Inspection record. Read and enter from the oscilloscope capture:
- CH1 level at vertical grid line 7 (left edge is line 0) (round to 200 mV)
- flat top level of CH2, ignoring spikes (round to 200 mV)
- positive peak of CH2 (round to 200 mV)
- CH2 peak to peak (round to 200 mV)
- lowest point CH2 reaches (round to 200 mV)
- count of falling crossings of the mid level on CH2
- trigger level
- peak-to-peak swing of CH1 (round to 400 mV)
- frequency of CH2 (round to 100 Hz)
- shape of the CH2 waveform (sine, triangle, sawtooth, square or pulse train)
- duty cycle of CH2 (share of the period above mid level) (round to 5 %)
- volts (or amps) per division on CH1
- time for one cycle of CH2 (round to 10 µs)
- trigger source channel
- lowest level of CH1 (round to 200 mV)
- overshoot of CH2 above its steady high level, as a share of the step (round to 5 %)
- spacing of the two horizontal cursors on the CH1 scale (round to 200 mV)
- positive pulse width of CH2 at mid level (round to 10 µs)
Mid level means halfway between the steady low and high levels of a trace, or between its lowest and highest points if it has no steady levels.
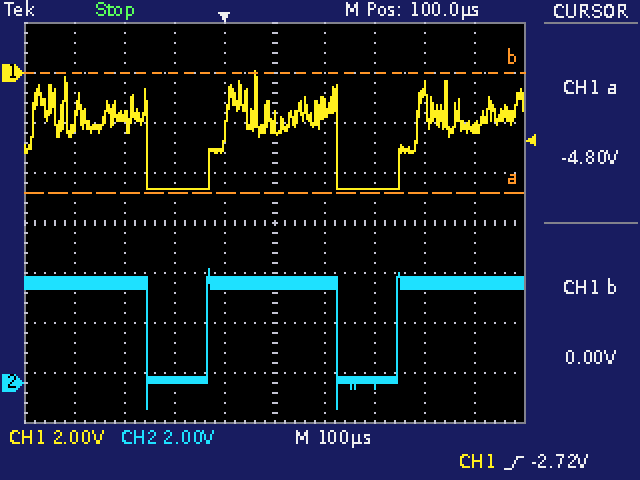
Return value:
-4.6 V
4.0 V
4.6 V
5.6 V
-1.0 V
2
-2.72 V
4.8 V
2.6 kHz
pulse train
70 %
2 V
380 µs
CH1
-4.6 V
15 %
4.8 V
260 µs
